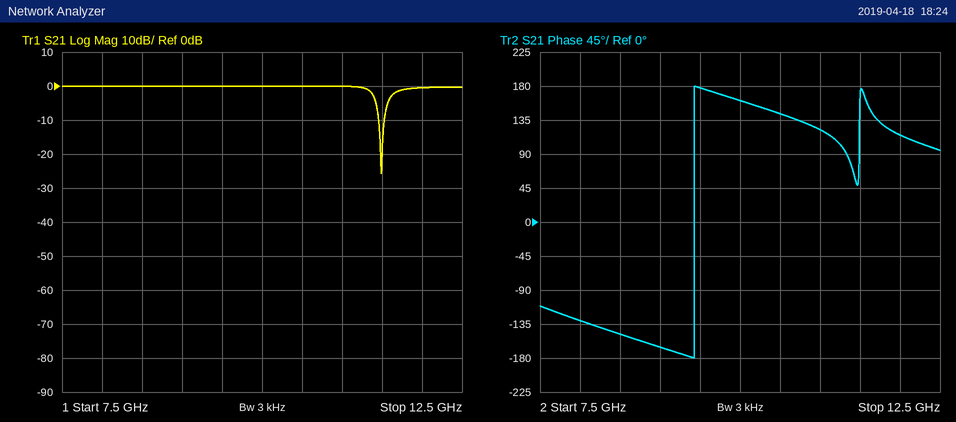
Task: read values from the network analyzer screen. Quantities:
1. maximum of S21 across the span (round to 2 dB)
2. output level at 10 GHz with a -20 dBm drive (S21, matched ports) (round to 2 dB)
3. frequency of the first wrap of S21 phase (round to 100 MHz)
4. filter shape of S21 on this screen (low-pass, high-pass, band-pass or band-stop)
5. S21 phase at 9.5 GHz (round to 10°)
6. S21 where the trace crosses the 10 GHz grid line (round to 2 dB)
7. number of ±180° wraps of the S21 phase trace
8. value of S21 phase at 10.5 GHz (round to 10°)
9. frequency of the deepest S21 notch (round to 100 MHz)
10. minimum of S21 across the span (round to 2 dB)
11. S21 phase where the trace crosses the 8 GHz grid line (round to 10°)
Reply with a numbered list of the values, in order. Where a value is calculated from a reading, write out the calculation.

1. 0 dB
2. -20 dBm + (0 dB) = -20 dBm
3. 9.4 GHz
4. band-stop
5. 180°
6. 0 dB
7. 1
8. 140°
9. 11.5 GHz
10. -26 dB
11. -130°
